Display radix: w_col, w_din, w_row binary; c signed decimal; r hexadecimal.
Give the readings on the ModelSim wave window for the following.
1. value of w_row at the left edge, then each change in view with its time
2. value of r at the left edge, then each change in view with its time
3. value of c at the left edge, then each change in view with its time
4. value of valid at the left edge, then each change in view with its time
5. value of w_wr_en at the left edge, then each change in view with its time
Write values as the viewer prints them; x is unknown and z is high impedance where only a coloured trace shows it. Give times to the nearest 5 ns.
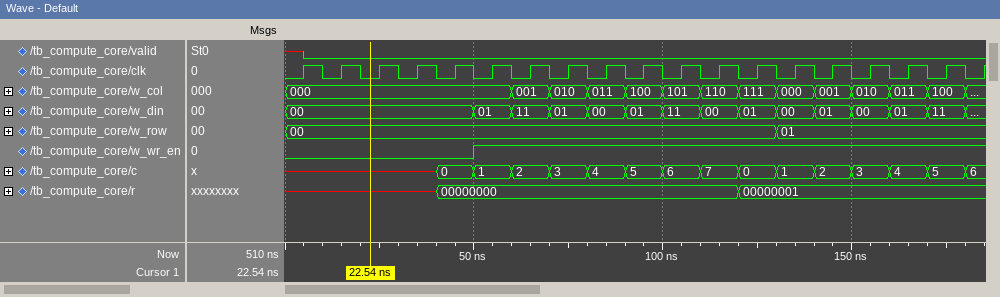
00, 01 at 130 ns
x, 00000000 at 40 ns, 00000001 at 120 ns
x, 0 at 40 ns, 1 at 50 ns, 2 at 60 ns, 3 at 70 ns, 4 at 80 ns, 5 at 90 ns, 6 at 100 ns, 7 at 110 ns, 0 at 120 ns, 1 at 130 ns, 2 at 140 ns, 3 at 150 ns, 4 at 160 ns, 5 at 170 ns, 6 at 180 ns
x, 0 at 5 ns
0, 1 at 50 ns
